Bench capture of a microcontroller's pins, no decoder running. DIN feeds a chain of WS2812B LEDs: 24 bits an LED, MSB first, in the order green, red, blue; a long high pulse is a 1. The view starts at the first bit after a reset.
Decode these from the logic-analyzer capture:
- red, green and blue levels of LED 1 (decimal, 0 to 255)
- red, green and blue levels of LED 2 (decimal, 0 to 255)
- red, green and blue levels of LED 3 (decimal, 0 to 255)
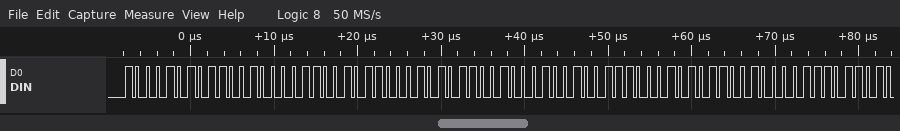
200, 138, 101
200, 138, 147
200, 138, 118
